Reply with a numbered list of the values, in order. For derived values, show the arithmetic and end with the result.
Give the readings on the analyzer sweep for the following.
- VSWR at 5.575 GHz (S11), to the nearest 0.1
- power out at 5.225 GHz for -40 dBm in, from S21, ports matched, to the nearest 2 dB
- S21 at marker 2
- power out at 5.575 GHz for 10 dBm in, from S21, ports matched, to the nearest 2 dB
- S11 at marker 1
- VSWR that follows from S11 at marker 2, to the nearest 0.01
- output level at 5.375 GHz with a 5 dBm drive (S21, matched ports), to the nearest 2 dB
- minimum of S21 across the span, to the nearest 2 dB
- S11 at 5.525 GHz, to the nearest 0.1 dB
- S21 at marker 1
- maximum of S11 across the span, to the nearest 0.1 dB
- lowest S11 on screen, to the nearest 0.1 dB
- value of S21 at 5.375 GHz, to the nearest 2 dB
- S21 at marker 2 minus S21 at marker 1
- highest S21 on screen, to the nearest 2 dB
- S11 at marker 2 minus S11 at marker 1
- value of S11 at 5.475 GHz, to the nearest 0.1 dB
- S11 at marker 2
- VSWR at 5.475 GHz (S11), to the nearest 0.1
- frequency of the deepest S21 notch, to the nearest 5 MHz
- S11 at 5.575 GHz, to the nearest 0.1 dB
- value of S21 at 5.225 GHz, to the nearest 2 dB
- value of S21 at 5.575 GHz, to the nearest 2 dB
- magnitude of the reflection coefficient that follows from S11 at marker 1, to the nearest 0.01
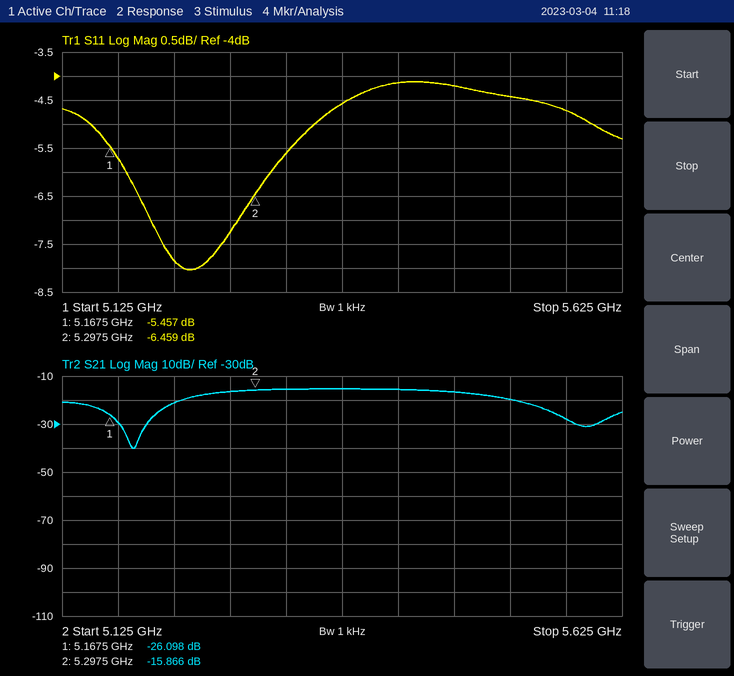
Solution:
1. |Γ| = 10^(-4.7/20) = 0.5821; VSWR = (1 + 0.5821)/(1 − 0.5821) ≈ 3.8
2. -40 dBm + (-22 dB) = -62 dBm
3. -15.866 dB
4. 10 dBm + (-28 dB) = -18 dBm
5. -5.457 dB
6. (1 + 0.4754)/(1 − 0.4754) ≈ 2.81
7. 5 dBm + (-16 dB) = -10 dBm
8. -40 dB
9. -4.4 dB
10. -26.098 dB
11. -4.1 dB
12. -8.0 dB
13. -16 dB
14. -15.866 − (-26.098) = 10.232 dB
15. -16 dB
16. -6.459 − (-5.457) = -1.002 dB
17. -4.2 dB
18. -6.459 dB
19. |Γ| = 10^(-4.2/20) = 0.6166; VSWR = (1 + 0.6166)/(1 − 0.6166) ≈ 4.2
20. 5.190 GHz
21. -4.7 dB
22. -22 dB
23. -28 dB
24. 10^(-5.457/20) ≈ 0.53
